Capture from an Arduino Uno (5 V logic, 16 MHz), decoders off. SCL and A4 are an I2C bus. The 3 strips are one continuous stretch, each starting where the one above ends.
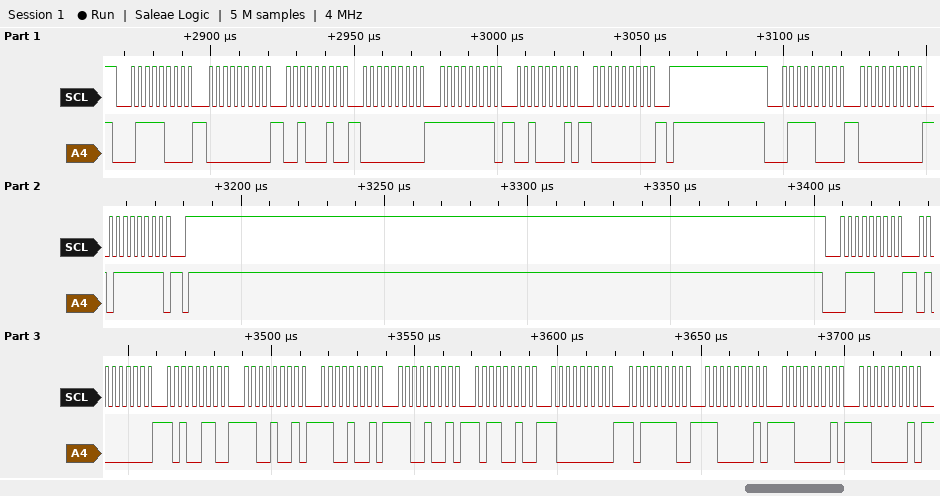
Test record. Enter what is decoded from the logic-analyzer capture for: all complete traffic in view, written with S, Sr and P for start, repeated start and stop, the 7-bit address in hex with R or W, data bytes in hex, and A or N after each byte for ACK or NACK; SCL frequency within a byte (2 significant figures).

S 3CW A 00 A 22 A 00 A FF A 21 A 00 A P S 3CW A 00 A 7F A P S 3CW A 40 A A6 A C9 A C9 A C9 A B2 A 80 A BE A C1 A C1 A C1 A
400 kHz
